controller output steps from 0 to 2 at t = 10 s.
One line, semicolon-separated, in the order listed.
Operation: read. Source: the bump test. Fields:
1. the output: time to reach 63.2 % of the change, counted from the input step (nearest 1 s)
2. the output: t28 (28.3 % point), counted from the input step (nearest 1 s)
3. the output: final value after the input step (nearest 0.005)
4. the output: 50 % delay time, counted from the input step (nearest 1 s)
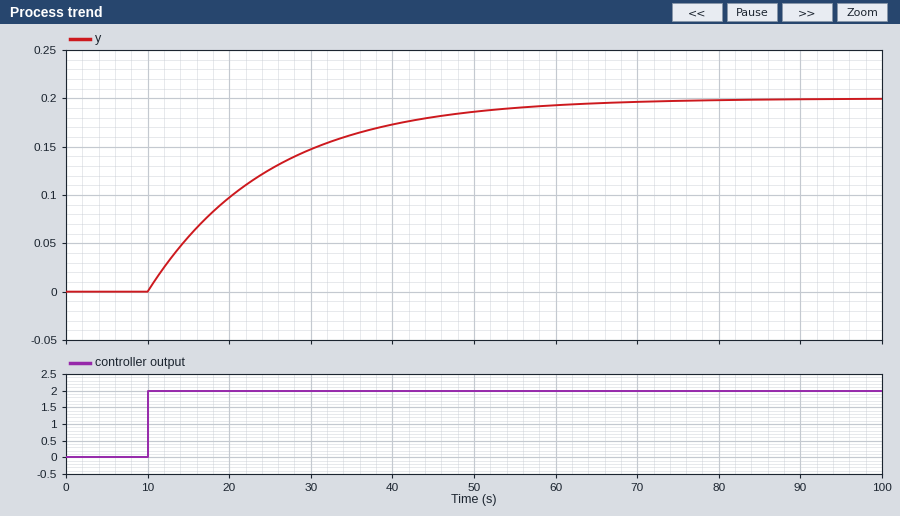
15 s; 5 s; 0.200; 10 s
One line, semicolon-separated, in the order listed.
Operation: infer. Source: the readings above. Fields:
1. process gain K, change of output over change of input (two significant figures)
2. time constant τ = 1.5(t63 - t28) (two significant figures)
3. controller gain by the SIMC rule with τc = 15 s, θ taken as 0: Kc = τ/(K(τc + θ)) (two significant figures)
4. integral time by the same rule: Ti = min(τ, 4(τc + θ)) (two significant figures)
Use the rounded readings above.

0.10; 15 s; 10; 15 s
